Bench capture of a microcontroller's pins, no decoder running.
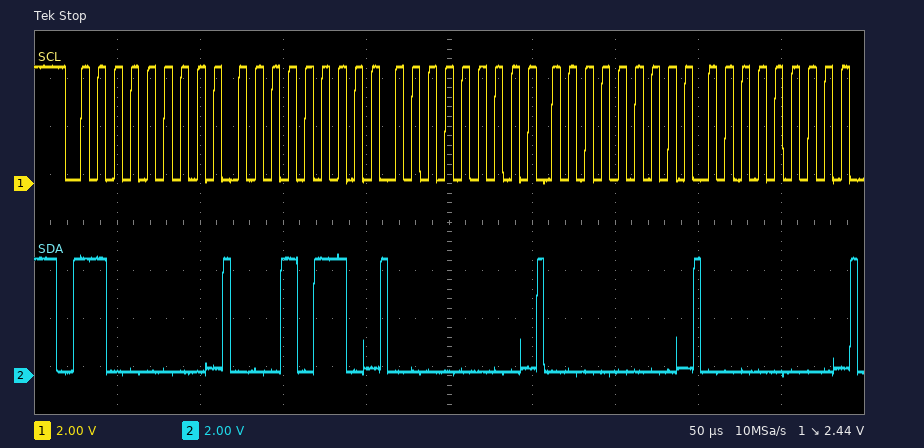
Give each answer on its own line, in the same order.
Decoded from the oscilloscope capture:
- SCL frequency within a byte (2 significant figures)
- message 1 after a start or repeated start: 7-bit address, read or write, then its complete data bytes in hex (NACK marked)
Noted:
100 kHz
0x60 write: 16 00 00 00
